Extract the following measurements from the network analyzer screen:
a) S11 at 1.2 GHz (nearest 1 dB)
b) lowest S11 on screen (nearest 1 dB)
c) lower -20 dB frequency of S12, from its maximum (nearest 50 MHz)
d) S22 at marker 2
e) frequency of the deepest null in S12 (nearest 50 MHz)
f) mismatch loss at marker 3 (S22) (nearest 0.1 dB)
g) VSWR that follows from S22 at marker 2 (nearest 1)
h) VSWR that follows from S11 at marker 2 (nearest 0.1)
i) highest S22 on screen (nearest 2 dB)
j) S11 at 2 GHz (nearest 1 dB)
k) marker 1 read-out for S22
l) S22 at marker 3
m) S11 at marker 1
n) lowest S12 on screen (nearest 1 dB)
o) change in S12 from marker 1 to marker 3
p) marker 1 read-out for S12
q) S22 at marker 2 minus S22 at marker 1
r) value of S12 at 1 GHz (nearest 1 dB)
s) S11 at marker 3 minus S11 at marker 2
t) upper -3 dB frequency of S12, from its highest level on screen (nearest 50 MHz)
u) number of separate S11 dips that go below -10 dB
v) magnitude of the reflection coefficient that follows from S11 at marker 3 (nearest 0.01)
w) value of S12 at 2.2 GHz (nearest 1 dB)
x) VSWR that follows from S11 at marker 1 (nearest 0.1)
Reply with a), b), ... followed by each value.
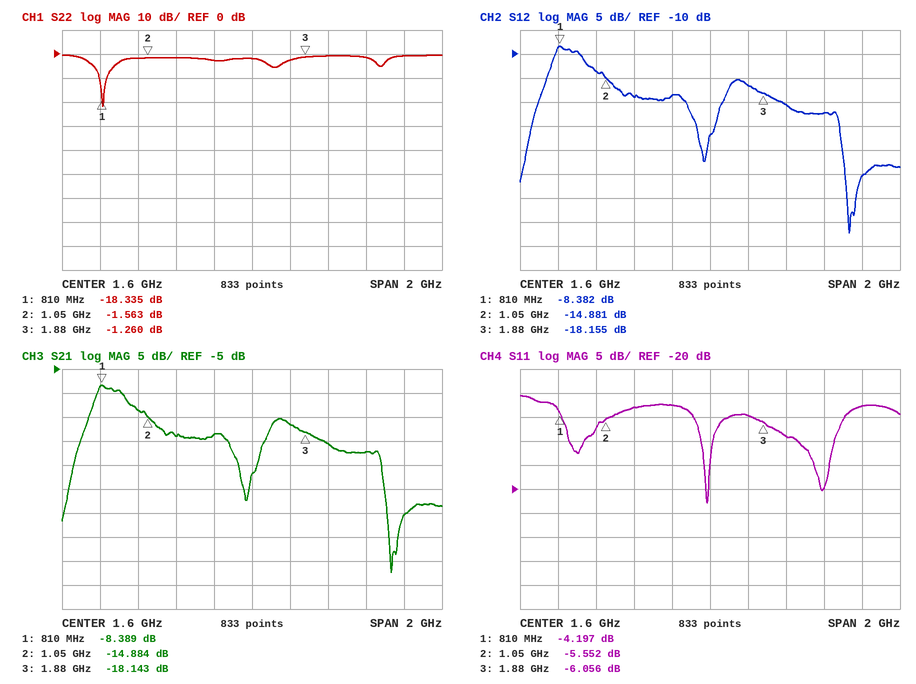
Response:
a) -3 dB
b) -23 dB
c) 650 MHz
d) -1.563 dB
e) 2.35 GHz
f) 6.0 dB
g) 11
h) 3.2
i) 0 dB
j) -9 dB
k) -18.335 dB
l) -1.260 dB
m) -4.197 dB
n) -47 dB
o) -9.773 dB
p) -8.382 dB
q) 16.772 dB
r) -14 dB
s) -0.504 dB
t) 950 MHz
u) 3
v) 0.50
w) -22 dB
x) 4.2
